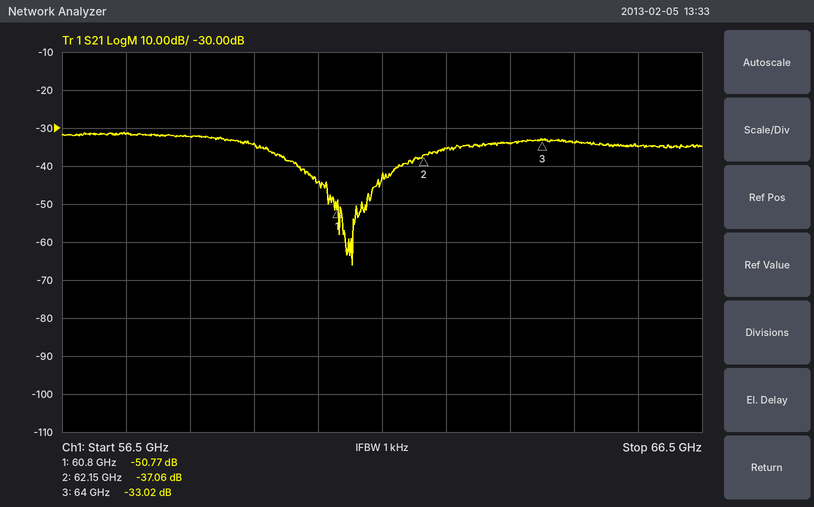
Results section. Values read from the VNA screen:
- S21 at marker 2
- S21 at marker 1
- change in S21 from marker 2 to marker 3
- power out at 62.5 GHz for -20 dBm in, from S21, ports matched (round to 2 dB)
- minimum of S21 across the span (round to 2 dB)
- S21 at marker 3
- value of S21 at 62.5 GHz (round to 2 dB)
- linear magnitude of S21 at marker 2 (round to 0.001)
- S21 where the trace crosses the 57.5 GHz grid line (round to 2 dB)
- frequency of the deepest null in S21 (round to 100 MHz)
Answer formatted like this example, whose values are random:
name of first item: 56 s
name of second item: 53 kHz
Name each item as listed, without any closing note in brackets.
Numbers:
S21 at marker 2: -37.06 dB
S21 at marker 1: -50.77 dB
change in S21 from marker 2 to marker 3: 4.04 dB
power out at 62.5 GHz for -20 dBm in, from S21, ports matched: -56 dBm
minimum of S21 across the span: -66 dB
S21 at marker 3: -33.02 dB
value of S21 at 62.5 GHz: -36 dB
linear magnitude of S21 at marker 2: 0.014
S21 where the trace crosses the 57.5 GHz grid line: -32 dB
frequency of the deepest null in S21: 61.0 GHz
